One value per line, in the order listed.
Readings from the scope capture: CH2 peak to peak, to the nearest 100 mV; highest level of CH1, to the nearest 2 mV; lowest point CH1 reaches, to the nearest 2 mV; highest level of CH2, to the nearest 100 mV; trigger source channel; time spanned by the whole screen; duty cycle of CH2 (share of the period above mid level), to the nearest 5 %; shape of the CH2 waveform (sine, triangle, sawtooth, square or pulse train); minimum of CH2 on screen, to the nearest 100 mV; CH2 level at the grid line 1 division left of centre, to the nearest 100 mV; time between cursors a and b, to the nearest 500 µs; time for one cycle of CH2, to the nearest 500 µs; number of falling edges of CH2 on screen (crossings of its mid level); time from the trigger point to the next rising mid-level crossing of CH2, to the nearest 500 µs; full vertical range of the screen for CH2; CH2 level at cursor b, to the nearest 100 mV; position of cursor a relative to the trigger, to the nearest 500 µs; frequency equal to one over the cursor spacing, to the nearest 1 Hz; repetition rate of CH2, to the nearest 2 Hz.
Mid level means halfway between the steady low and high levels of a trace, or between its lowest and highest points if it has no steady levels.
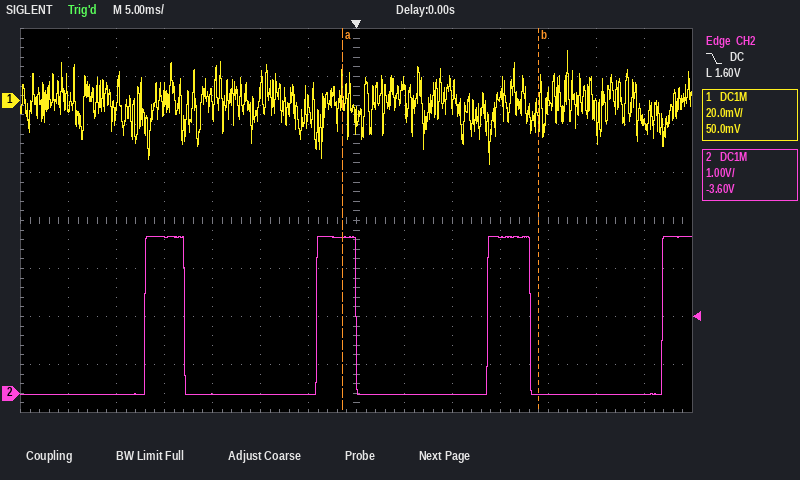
3.3 V
20 mV
-26 mV
3.3 V
CH2
70 ms
25 %
pulse train
0.0 V
0.0 V
20.5 ms
18.0 ms
3
13.5 ms
8 V
0.0 V
-1.5 ms
49 Hz
56 Hz
